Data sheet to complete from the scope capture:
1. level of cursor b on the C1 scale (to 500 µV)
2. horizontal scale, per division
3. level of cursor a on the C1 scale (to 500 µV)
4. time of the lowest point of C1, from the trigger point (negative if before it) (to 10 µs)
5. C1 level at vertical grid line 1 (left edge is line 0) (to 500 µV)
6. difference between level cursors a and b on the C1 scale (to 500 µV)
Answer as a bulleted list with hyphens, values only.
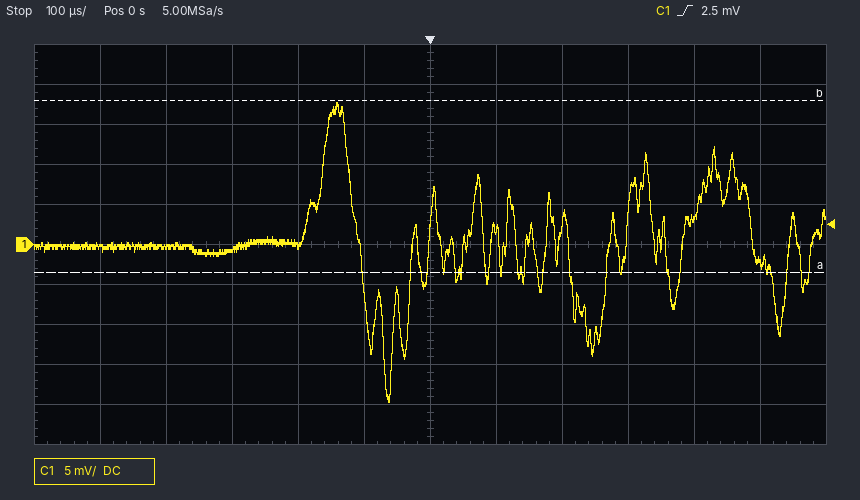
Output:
- 18.0 mV
- 100 µs
- -3.5 mV
- -60 µs
- -500 µV
- 21.5 mV
